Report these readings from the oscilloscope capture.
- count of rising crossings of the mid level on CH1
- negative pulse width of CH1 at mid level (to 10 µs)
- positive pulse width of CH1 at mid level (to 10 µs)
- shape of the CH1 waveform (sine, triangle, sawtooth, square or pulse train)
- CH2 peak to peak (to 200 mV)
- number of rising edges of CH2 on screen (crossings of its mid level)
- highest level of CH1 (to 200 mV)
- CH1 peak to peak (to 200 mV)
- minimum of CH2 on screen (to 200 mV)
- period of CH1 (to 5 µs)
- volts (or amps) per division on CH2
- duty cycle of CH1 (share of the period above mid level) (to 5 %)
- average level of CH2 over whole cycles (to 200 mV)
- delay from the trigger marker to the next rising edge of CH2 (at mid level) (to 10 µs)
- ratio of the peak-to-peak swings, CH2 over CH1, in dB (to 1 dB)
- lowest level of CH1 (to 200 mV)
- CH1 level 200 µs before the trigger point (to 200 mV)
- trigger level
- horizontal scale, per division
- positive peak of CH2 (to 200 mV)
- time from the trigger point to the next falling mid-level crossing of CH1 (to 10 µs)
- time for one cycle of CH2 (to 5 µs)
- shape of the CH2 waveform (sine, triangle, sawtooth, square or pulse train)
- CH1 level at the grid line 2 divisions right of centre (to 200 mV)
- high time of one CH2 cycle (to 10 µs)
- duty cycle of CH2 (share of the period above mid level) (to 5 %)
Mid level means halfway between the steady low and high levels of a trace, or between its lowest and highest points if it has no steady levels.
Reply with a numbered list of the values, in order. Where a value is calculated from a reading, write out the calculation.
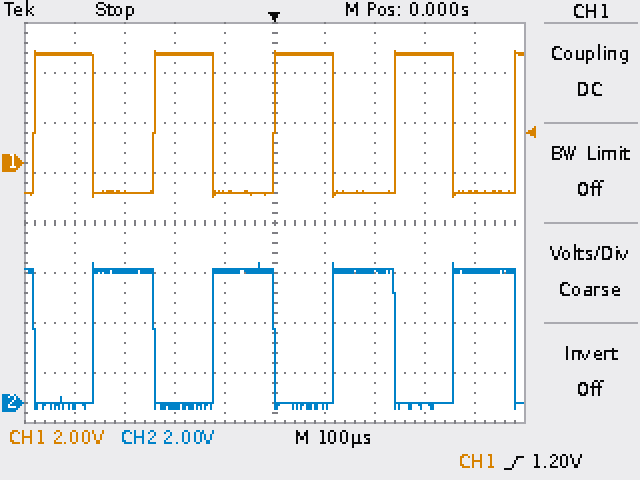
1. 5
2. 120 µs
3. 120 µs
4. square
5. 5.6 V − (-200 mV) = 5.8 V
6. 4
7. 4.4 V
8. 4.4 V − (-1.4 V) = 5.8 V
9. -200 mV
10. 240 µs
11. 2 V
12. 120 µs / 240 µs ≈ 50 %
13. -200 mV + 0.5 × (5.6 V − (-200 mV)) ≈ 2.70 V, so 2.8 V to the nearest 200 mV
14. 120 µs
15. 20 log10(5.8 V / 5.8 V) ≈ 0 dB
16. -1.4 V
17. 4.4 V
18. 1.20 V
19. 100 µs
20. 5.6 V
21. 120 µs
22. 240 µs
23. square
24. -1.2 V
25. 120 µs
26. 120 µs / 240 µs ≈ 50 %
